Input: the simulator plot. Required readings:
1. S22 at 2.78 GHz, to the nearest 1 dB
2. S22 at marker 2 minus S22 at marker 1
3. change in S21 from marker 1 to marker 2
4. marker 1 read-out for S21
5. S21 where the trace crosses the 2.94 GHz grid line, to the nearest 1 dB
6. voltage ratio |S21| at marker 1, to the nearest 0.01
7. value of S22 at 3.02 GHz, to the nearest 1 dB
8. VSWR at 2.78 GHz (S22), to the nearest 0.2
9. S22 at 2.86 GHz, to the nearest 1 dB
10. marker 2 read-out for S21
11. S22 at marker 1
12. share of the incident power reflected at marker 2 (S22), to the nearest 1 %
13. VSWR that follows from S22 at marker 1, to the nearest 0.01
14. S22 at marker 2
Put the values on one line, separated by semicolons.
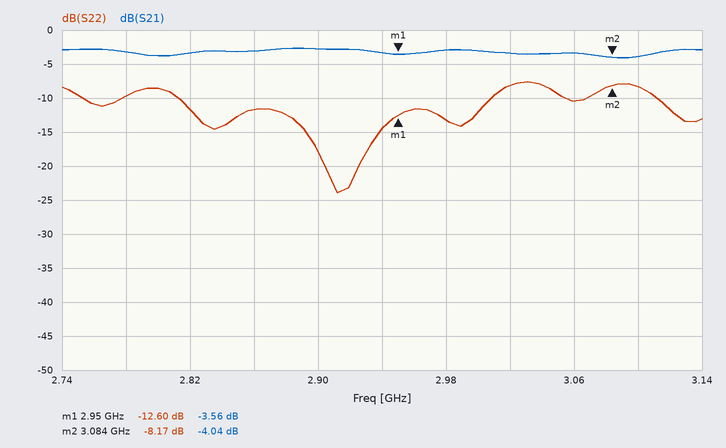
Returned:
-10 dB; 4.43 dB; -0.48 dB; -3.56 dB; -3 dB; 0.66; -8 dB; 2.0; -12 dB; -4.04 dB; -12.60 dB; 15 %; 1.61; -8.17 dB
